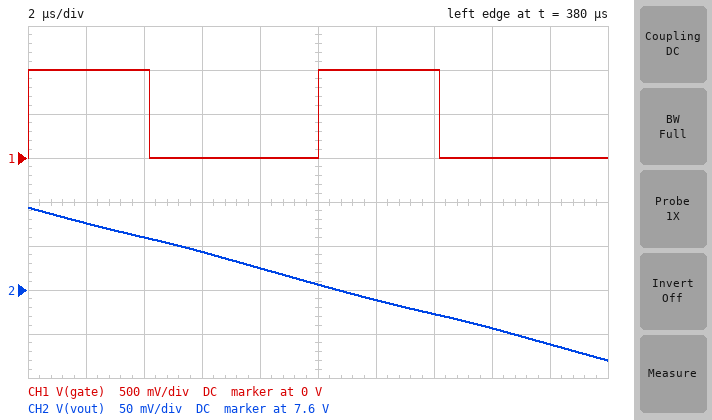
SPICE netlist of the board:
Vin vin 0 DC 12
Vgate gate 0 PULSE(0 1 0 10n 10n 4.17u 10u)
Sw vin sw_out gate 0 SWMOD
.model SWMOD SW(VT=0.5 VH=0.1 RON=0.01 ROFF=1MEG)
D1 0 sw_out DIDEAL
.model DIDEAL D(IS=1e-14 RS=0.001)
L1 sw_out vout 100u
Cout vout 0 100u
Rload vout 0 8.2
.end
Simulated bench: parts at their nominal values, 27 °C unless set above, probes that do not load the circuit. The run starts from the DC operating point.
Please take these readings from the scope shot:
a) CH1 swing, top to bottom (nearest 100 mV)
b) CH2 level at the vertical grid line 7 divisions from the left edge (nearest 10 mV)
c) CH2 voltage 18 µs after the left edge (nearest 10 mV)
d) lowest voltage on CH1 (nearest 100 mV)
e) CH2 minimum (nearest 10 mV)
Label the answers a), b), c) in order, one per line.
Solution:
a) 1.0 V
b) 7.57 V
c) 7.54 V
d) 0 V
e) 7.52 V
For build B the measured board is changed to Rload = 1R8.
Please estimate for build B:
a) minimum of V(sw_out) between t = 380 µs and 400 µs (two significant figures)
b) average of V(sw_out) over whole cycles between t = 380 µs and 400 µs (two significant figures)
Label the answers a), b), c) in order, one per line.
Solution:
a) -860 mV
b) 4.5 V
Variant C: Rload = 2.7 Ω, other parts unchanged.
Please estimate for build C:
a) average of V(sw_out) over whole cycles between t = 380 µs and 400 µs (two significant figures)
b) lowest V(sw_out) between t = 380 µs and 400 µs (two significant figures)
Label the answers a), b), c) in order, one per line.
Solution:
a) 4.5 V
b) -840 mV
